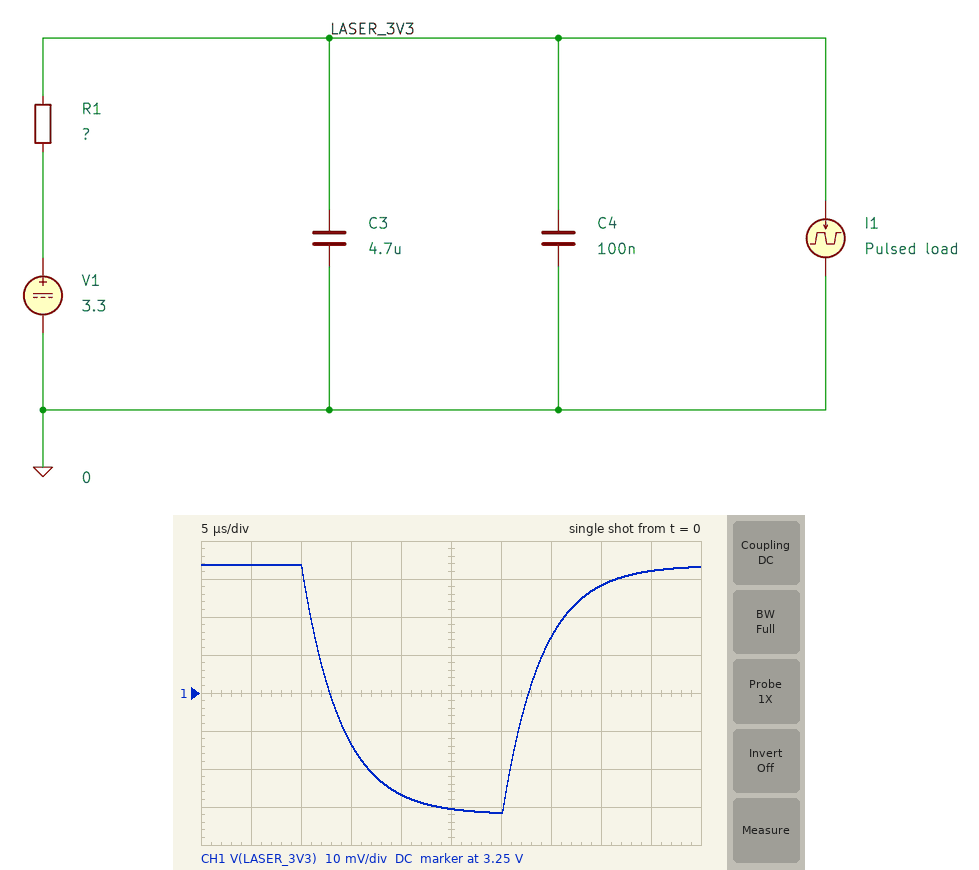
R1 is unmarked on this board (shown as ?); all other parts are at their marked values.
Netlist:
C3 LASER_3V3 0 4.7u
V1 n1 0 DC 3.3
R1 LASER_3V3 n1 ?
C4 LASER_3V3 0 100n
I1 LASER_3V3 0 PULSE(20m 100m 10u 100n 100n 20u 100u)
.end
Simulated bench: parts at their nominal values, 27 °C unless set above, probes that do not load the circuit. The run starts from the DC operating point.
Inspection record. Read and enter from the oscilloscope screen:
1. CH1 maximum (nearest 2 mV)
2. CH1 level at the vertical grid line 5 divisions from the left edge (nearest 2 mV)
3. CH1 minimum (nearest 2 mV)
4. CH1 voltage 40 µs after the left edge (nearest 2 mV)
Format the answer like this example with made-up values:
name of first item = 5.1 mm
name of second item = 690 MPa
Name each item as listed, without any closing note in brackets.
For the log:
CH1 maximum = 3.284 V
CH1 level at the vertical grid line 5 divisions from the left edge = 3.220 V
CH1 minimum = 3.218 V
CH1 voltage 40 µs after the left edge = 3.278 V
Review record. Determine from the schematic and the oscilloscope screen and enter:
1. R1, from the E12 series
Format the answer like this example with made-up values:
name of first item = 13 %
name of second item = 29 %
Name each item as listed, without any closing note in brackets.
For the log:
R1, from the E12 series = 0.82 Ω
